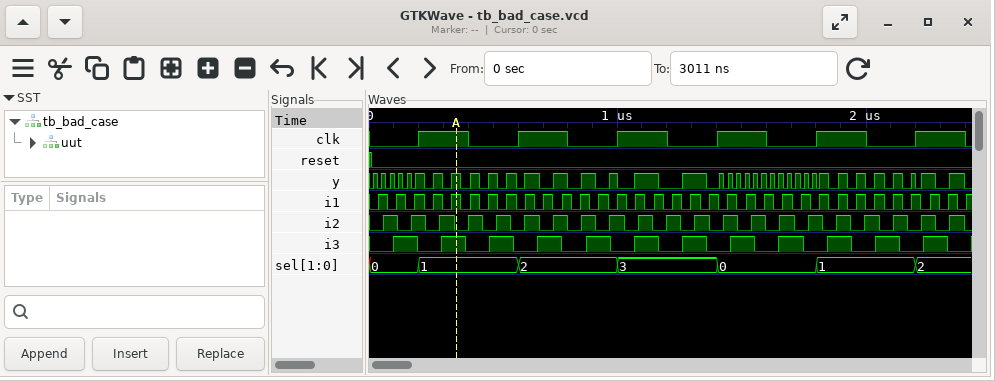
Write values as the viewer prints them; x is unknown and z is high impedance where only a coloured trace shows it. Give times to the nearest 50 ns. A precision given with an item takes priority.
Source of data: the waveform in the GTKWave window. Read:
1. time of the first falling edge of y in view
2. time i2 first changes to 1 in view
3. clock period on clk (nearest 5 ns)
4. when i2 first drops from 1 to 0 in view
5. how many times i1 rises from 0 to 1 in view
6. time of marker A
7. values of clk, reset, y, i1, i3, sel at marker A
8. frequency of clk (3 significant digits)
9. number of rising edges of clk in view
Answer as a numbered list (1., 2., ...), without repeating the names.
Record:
1. 50 ns
2. 50 ns
3. 400 ns
4. 100 ns
5. 33
6. 350 ns
7. clk=1, reset=0, y=1, i1=1, i3=1, sel=1
8. 2.50 MHz
9. 6
